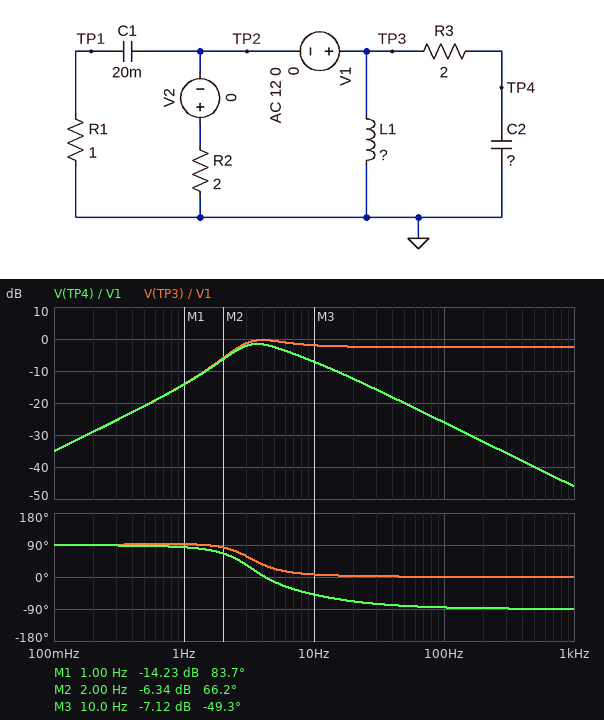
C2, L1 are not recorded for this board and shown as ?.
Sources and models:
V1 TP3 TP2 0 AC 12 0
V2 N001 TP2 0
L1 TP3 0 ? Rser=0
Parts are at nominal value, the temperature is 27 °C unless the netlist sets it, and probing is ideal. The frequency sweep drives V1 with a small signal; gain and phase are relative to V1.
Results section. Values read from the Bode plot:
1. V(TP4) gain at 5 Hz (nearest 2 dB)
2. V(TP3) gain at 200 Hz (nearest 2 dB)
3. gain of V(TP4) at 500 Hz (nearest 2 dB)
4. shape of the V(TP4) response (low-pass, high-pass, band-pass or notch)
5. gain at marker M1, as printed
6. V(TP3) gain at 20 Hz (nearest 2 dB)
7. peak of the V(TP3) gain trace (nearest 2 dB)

-2 dB
-2 dB
-40 dB
band-pass
-14.23 dB
-2 dB
0 dB
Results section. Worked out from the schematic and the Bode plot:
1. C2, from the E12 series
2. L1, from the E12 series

12 mF
56 mH
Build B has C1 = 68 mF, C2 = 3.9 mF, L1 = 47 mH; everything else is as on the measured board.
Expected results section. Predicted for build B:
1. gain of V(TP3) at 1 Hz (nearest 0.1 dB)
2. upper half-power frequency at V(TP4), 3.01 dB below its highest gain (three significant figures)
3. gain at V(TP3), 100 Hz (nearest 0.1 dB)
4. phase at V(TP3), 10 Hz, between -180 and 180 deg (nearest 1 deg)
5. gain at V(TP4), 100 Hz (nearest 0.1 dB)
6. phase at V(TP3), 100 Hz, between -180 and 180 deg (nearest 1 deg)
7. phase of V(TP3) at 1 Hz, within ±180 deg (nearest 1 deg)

-12.3 dB
15.7 Hz
-2.4 dB
6 deg
-16.4 dB
-2 deg
107 deg
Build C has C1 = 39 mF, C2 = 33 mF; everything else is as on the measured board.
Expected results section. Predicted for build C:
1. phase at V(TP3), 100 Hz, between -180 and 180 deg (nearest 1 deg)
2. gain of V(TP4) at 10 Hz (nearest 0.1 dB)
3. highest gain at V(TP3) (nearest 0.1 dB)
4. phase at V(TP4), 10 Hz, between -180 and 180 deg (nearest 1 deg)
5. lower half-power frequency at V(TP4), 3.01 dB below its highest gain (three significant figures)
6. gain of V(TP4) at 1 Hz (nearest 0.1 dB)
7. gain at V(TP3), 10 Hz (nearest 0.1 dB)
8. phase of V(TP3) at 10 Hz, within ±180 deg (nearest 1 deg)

1 deg
-15.0 dB
-1.6 dB
-68 deg
1.52 Hz
-13.1 dB
-2.4 dB
9 deg
